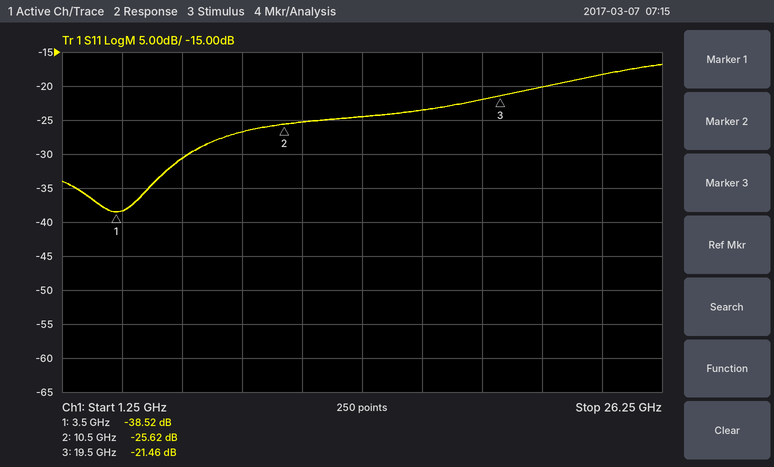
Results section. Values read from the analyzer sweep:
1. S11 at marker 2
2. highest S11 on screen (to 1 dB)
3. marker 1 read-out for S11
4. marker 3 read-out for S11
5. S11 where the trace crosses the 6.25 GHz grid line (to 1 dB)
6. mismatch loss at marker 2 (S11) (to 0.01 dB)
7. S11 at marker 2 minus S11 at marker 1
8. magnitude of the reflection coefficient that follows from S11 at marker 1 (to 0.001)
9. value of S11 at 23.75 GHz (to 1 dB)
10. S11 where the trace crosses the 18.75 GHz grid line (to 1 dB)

-25.62 dB
-17 dB
-38.52 dB
-21.46 dB
-31 dB
0.01 dB
12.90 dB
0.012
-18 dB
-22 dB
